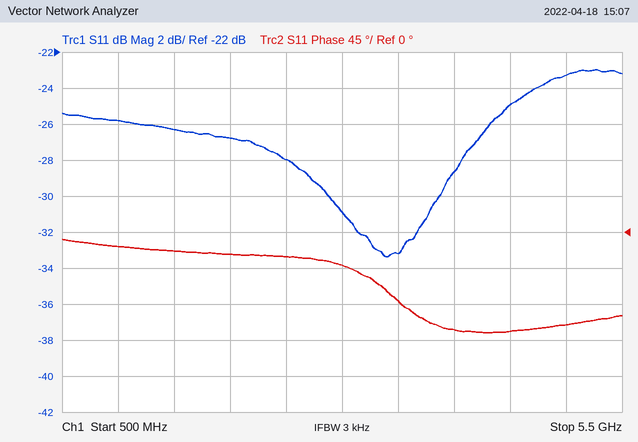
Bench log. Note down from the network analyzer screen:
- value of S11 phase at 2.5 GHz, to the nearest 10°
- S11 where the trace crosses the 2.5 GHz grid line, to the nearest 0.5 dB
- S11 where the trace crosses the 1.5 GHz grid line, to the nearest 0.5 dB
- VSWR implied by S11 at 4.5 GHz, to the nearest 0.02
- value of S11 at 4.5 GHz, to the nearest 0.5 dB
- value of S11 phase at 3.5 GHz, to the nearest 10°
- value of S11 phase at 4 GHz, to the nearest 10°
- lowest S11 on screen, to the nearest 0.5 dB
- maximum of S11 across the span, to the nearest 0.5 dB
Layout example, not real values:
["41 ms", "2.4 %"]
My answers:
["-30°", "-28.0 dB", "-26.5 dB", "1.12", "-25.0 dB", "-90°", "-120°", "-33.5 dB", "-23.0 dB"]
